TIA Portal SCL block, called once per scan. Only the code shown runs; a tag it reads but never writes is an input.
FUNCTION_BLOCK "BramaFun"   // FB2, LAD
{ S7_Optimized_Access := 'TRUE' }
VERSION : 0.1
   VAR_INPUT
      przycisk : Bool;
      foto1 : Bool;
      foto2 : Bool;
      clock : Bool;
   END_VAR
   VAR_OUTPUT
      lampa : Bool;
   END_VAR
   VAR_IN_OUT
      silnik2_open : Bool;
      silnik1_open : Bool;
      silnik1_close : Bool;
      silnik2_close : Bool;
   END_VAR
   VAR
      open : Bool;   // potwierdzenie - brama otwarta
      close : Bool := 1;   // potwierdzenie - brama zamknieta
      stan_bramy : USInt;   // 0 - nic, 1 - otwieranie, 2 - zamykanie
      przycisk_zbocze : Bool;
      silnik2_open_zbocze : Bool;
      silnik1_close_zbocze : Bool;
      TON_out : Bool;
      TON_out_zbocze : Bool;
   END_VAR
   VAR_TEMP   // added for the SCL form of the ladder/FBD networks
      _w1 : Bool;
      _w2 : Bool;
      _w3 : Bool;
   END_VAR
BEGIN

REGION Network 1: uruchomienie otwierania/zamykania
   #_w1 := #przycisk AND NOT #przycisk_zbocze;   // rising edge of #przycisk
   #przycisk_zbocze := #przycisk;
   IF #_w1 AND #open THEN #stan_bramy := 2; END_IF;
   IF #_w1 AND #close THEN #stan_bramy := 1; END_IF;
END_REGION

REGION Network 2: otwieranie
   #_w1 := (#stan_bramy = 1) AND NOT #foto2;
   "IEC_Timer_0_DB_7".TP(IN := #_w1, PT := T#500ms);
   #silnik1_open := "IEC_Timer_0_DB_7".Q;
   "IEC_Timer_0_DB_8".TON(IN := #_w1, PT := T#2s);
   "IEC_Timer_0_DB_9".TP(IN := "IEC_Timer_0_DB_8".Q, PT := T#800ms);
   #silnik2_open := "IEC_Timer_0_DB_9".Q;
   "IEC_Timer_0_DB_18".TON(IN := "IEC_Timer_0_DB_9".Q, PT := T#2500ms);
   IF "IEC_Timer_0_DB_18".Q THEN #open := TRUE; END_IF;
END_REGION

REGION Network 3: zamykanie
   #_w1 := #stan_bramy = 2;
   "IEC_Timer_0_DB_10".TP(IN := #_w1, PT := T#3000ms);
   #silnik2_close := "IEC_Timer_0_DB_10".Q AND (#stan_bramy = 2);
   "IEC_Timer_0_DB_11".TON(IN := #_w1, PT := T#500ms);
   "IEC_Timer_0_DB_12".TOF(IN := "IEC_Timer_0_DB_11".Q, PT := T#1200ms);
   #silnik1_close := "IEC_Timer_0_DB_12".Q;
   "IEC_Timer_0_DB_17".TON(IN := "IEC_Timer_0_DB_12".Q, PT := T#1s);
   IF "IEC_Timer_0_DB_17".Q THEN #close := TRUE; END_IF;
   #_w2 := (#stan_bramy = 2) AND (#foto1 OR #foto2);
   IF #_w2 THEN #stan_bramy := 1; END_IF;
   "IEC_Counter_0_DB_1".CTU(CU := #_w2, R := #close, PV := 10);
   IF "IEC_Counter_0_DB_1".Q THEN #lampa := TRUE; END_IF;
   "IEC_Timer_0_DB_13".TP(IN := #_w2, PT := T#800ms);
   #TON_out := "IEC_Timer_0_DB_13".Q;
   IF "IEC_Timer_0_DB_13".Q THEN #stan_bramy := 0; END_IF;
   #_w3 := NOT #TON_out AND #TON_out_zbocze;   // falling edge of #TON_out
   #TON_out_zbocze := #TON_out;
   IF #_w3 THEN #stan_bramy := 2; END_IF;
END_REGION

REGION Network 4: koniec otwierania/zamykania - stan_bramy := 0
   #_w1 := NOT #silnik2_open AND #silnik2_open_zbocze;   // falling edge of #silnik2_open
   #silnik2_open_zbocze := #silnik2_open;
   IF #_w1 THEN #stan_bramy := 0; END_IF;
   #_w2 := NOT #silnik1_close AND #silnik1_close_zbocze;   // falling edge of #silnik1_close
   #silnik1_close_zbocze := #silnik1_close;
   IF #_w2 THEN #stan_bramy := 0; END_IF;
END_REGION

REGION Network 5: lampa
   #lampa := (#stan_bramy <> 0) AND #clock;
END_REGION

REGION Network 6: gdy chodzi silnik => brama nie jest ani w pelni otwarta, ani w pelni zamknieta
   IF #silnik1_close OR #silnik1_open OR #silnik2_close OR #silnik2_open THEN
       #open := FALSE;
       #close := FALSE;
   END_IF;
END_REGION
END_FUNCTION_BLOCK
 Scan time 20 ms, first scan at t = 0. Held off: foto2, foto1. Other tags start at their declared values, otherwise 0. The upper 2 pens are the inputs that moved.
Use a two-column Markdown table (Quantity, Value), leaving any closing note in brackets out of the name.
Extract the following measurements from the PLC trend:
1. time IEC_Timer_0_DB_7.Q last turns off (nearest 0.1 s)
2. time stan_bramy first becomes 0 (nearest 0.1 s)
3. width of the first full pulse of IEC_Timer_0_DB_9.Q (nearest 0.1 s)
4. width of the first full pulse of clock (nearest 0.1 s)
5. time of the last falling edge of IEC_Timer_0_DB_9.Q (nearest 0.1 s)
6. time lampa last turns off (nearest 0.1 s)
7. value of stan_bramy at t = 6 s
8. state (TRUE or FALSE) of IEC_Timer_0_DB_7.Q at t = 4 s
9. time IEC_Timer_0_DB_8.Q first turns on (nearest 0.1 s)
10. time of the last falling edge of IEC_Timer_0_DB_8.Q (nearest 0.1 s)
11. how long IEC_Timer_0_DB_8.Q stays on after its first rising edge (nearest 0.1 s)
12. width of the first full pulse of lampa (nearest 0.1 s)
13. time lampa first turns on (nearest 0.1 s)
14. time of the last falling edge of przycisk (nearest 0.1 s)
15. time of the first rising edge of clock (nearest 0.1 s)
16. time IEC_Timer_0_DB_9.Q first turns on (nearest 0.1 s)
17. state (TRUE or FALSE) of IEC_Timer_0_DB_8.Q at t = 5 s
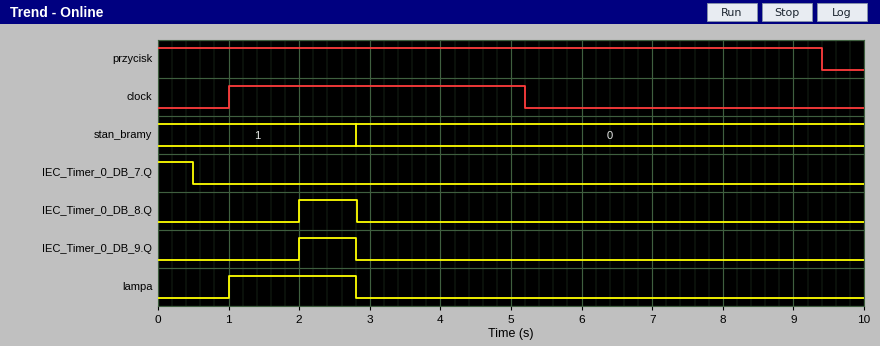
| Quantity | Value |
|---|---|
| time IEC_Timer_0_DB_7.Q last turns off | 0.5 s |
| time stan_bramy first becomes 0 | 2.8 s |
| width of the first full pulse of IEC_Timer_0_DB_9.Q | 0.8 s |
| width of the first full pulse of clock | 4.2 s |
| time of the last falling edge of IEC_Timer_0_DB_9.Q | 2.8 s |
| time lampa last turns off | 2.8 s |
| value of stan_bramy at t = 6 s | 0 |
| state (TRUE or FALSE) of IEC_Timer_0_DB_7.Q at t = 4 s | FALSE |
| time IEC_Timer_0_DB_8.Q first turns on | 2.0 s |
| time of the last falling edge of IEC_Timer_0_DB_8.Q | 2.8 s |
| how long IEC_Timer_0_DB_8.Q stays on after its first rising edge | 0.8 s |
| width of the first full pulse of lampa | 1.8 s |
| time lampa first turns on | 1.0 s |
| time of the last falling edge of przycisk | 9.4 s |
| time of the first rising edge of clock | 1.0 s |
| time IEC_Timer_0_DB_9.Q first turns on | 2.0 s |
| state (TRUE or FALSE) of IEC_Timer_0_DB_8.Q at t = 5 s | FALSE |
